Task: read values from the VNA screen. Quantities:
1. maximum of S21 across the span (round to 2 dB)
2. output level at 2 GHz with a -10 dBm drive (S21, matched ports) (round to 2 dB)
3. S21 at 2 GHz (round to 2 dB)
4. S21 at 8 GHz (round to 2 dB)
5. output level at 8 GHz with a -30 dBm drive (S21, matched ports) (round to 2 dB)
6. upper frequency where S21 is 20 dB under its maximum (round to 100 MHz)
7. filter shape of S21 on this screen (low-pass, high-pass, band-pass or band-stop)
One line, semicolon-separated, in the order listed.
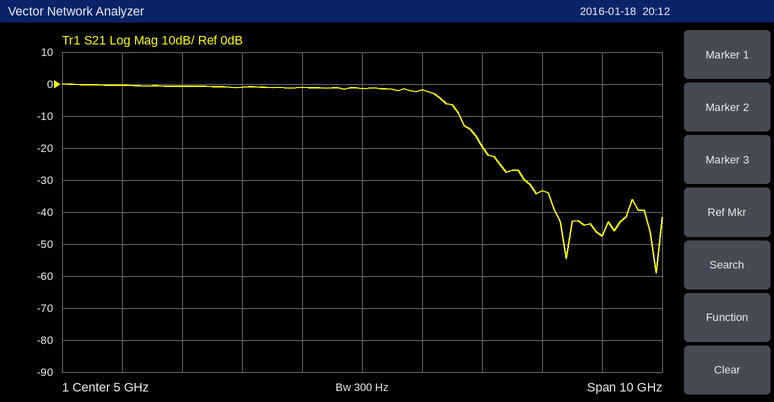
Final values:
0 dB; -10 dBm; 0 dB; -34 dB; -64 dBm; 7.0 GHz; low-pass
